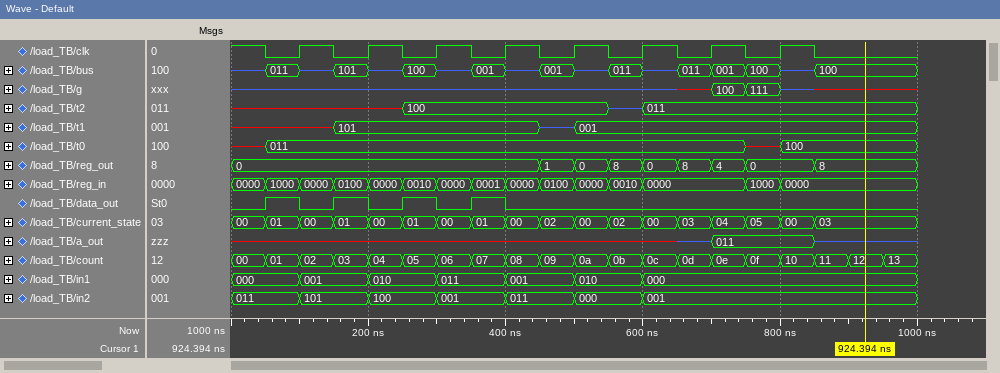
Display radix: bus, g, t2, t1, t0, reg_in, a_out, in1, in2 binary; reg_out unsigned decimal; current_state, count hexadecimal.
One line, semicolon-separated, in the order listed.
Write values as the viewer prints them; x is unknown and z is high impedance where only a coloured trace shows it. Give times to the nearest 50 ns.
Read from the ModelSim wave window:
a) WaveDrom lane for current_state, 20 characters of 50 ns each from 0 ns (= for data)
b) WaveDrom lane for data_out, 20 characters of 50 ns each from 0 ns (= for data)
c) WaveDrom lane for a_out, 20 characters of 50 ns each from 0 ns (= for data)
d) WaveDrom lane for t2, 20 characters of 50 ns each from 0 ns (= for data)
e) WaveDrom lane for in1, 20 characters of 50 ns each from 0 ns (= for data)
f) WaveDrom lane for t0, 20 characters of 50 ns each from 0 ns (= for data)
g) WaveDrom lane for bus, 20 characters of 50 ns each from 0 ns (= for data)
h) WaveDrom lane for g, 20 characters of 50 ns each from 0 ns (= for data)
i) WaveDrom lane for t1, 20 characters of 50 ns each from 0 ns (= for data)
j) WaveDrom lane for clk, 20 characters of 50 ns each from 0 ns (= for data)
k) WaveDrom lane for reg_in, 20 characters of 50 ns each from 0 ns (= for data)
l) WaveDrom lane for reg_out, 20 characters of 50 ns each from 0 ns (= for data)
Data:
{name: 'current_state', wave: '==================..', data: '00 01 00 01 00 01 00 01 00 02 00 02 00 03 04 05 00 03'}; {name: 'data_out', wave: '010101010...........'}; {name: 'a_out', wave: 'x............z=..z..', data: '011'}; {name: 't2', wave: 'x....=.....z=.......', data: '100 011'}; {name: 'in1', wave: '=.=.=.=.=.=.=.......', data: '000 001 010 011 001 010 000'}; {name: 't0', wave: 'x=.............x=...', data: '011 100'}; {name: 'bus', wave: 'z=z=z=z=z=z=z===z=..', data: '011 101 100 001 001 011 011 001 100 100'}; {name: 'g', wave: 'z............x==zx..', data: '100 111'}; {name: 't1', wave: 'x..=.....z=.........', data: '101 001'}; {name: 'clk', wave: '101010101010101010..'}; {name: 'reg_in', wave: '=============..==...', data: '0000 1000 0000 0100 0000 0010 0000 0001 0000 0100 0000 0010 0000 1000 0000'}; {name: 'reg_out', wave: '=........=======.=..', data: '0 1 0 8 0 8 4 0 8'}
